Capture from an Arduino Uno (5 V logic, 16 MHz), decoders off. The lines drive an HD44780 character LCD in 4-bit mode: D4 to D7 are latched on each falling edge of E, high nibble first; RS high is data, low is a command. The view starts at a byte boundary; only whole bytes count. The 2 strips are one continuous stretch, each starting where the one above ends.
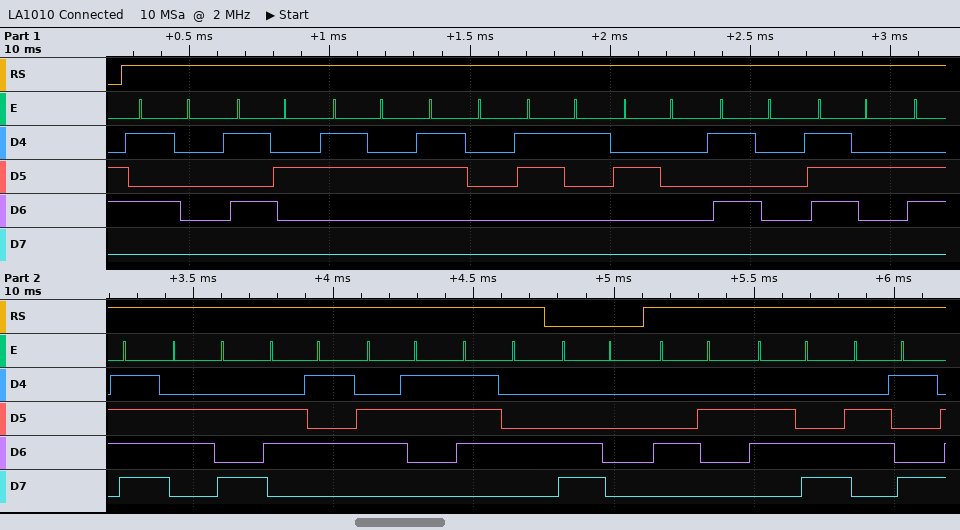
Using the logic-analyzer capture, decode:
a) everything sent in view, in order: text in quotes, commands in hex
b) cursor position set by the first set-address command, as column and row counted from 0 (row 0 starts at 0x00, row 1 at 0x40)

"PR201 Project" 0xC0 "Bli"
column 0, row 1
